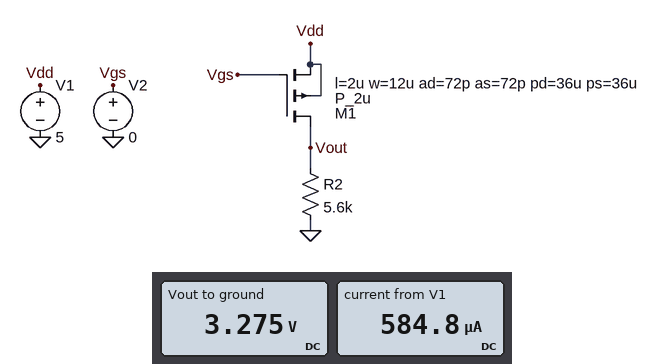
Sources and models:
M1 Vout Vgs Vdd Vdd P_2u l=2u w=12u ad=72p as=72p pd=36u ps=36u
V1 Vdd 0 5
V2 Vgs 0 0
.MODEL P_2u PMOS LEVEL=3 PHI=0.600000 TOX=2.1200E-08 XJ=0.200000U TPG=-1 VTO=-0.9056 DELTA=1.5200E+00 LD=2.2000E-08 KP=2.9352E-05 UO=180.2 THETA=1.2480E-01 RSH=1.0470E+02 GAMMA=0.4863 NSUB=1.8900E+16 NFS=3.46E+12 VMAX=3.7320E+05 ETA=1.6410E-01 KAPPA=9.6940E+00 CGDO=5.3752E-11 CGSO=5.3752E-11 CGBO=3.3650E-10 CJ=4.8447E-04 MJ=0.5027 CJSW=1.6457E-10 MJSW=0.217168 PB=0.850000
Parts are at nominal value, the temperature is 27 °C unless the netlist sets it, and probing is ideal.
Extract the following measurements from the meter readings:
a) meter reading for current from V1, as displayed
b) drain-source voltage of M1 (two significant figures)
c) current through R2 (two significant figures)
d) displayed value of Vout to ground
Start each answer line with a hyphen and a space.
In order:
- 584.8 µA
- -1.7 V
- 580 µA
- 3.275 V
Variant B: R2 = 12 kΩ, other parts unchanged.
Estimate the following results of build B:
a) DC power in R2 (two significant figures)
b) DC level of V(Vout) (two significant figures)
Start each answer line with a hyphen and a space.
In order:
- 1.4 mW
- 4.1 V
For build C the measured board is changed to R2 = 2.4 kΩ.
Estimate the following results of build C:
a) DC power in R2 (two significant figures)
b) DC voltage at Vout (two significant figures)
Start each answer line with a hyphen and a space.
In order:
- 1.5 mW
- 1.9 V
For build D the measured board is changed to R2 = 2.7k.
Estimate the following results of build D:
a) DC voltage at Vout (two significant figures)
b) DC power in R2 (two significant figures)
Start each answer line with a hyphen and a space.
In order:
- 2.1 V
- 1.6 mW
